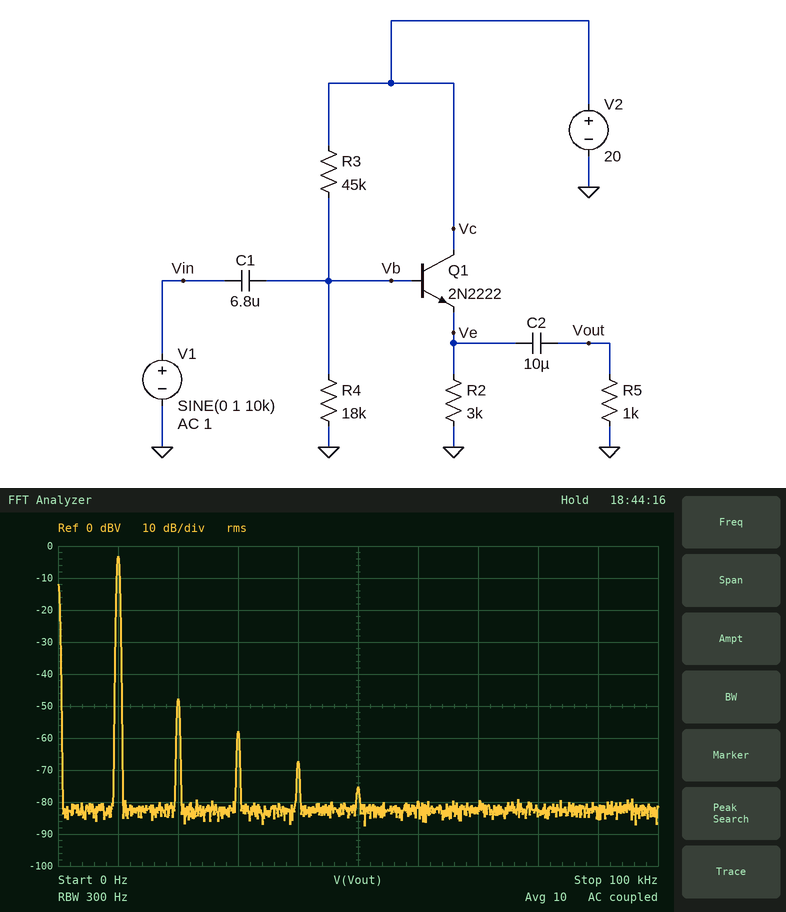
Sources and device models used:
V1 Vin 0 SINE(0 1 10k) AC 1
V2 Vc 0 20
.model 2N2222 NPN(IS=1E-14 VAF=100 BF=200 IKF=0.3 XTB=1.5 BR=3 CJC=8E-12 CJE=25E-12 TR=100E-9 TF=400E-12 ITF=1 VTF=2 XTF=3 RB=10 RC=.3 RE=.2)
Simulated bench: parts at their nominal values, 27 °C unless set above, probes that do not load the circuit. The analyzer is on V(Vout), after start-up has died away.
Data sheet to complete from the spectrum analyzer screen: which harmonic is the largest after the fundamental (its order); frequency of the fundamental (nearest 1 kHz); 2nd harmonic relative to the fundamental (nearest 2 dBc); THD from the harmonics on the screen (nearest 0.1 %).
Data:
2
10 kHz
-44 dBc
0.6 %
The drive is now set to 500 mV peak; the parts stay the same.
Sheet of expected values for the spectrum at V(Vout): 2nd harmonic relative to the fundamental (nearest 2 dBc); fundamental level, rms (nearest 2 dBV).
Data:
-54 dBc
-10 dBV
